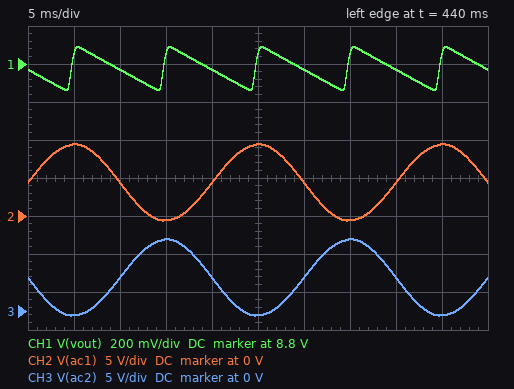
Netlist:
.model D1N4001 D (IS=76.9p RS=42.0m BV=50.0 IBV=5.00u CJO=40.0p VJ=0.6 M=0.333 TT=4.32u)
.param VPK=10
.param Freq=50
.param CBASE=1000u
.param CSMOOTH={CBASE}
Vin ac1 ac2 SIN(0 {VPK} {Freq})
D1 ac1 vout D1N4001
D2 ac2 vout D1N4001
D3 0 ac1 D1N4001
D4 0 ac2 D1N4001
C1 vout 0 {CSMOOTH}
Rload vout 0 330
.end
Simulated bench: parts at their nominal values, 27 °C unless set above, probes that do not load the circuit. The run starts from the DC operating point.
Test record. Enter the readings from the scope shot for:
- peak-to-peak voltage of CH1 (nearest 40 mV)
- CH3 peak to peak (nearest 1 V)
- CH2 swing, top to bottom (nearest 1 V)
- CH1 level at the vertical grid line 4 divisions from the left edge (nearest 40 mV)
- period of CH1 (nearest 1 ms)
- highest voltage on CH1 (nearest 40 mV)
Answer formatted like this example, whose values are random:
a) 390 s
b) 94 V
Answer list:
a) 240 mV
b) 10 V
c) 10 V
d) 8.76 V
e) 10 ms
f) 8.88 V
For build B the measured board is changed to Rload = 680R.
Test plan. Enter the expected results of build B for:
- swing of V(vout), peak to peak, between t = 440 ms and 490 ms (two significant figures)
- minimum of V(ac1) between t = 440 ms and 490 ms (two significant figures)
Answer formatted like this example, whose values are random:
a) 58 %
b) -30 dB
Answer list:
a) 110 mV
b) -570 mV
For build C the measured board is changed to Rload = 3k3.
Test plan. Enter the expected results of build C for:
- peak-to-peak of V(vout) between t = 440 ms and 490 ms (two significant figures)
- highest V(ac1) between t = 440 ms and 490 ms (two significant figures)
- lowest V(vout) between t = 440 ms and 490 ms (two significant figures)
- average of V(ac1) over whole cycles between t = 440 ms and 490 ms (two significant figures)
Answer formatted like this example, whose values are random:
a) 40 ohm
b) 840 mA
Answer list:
a) 24 mV
b) 9.5 V
c) 8.9 V
d) 4.5 V
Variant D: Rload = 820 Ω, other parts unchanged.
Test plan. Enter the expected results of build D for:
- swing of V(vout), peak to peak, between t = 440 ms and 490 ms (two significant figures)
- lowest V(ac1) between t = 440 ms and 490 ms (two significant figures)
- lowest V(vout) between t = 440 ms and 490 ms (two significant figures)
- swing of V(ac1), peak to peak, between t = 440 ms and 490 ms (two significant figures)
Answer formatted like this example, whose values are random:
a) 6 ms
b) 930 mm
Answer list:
a) 94 mV
b) -560 mV
c) 8.8 V
d) 10 V
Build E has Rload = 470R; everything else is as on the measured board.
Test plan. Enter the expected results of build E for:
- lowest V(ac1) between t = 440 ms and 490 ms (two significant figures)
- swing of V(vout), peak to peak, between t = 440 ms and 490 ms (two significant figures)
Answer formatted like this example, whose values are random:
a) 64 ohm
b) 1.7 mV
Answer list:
a) -580 mV
b) 160 mV
